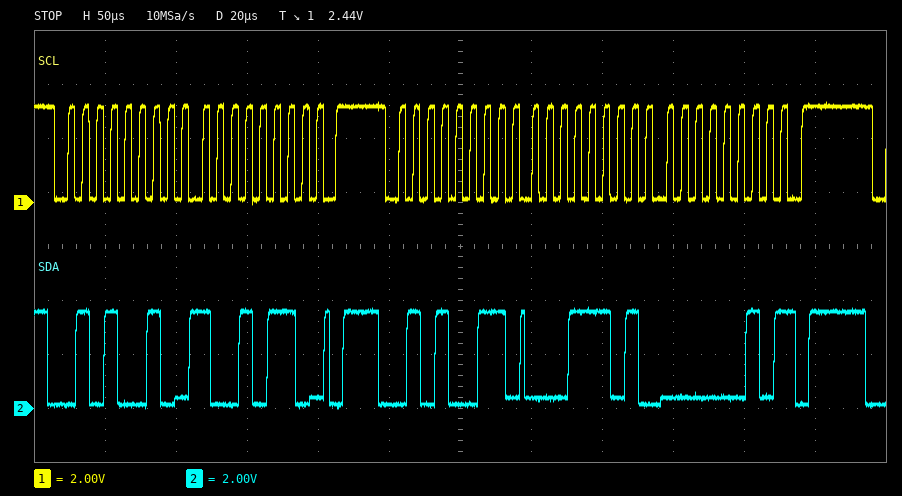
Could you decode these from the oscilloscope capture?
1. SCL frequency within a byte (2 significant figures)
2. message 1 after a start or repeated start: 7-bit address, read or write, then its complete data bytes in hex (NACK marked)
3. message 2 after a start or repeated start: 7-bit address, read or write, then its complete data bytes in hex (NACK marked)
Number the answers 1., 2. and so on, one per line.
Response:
1. 100 kHz
2. 0x29 write: 96
3. 0x29 read: 1D 02 NACK
